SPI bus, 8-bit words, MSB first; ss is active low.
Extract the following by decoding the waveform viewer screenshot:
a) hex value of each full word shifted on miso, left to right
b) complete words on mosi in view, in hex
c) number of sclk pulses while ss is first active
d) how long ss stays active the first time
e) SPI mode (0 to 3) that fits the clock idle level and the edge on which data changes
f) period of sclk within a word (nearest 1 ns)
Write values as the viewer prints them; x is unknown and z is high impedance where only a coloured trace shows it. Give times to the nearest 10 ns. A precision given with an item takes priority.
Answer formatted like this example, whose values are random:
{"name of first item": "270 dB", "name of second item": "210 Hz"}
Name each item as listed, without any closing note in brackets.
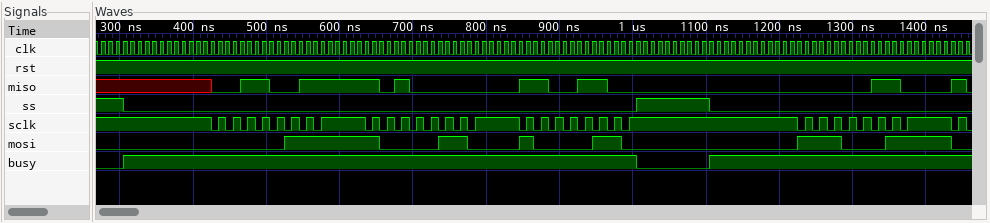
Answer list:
{"hex value of each full word shifted on miso, left to right": "33, A0, CC, 06", "complete words on mosi in view, in hex": "07, 86, 86, E3", "number of sclk pulses while ss is first active": "24", "how long ss stays active the first time": "700 ns", "SPI mode (0 to 3) that fits the clock idle level and the edge on which data changes": "3", "period of sclk within a word": "20 ns"}
